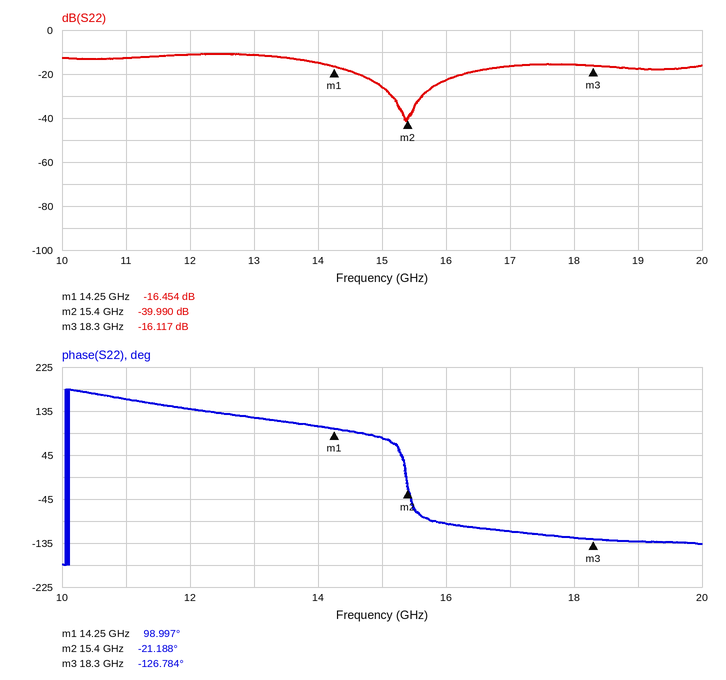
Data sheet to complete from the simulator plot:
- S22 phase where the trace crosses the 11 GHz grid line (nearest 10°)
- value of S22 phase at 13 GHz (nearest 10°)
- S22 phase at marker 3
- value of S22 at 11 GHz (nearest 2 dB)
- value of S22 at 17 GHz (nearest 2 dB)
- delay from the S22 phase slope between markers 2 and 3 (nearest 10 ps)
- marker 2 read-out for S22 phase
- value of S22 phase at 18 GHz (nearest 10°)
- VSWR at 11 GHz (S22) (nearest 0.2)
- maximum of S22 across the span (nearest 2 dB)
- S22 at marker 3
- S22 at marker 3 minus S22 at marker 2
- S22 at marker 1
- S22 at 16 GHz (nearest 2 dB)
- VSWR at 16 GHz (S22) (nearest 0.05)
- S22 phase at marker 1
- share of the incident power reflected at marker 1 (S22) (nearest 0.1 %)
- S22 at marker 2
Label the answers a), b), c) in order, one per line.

a) 160°
b) 120°
c) -126.784°
d) -12 dB
e) -16 dB
f) 100 ps
g) -21.188°
h) -120°
i) 1.6
j) -10 dB
k) -16.117 dB
l) 23.873 dB
m) -16.454 dB
n) -22 dB
o) 1.15
p) 98.997°
q) 2.3 %
r) -39.990 dB
